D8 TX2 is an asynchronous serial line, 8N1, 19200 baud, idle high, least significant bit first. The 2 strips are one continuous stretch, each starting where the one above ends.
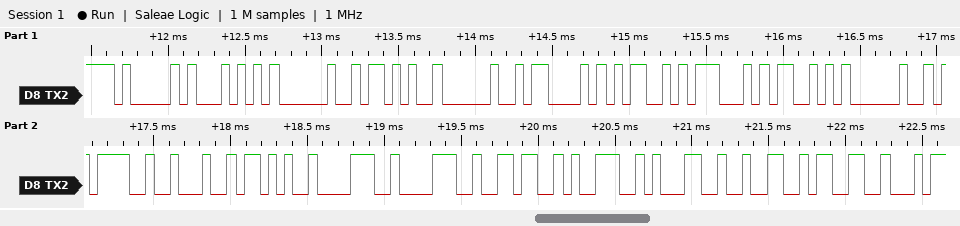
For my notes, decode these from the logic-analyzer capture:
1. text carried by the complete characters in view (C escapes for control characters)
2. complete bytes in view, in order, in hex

"AT + CMGS =\"+8869123"
41 54 20 2B 20 43 4D 47 53 20 3D 22 2B 38 38 36 39 31 32 33
